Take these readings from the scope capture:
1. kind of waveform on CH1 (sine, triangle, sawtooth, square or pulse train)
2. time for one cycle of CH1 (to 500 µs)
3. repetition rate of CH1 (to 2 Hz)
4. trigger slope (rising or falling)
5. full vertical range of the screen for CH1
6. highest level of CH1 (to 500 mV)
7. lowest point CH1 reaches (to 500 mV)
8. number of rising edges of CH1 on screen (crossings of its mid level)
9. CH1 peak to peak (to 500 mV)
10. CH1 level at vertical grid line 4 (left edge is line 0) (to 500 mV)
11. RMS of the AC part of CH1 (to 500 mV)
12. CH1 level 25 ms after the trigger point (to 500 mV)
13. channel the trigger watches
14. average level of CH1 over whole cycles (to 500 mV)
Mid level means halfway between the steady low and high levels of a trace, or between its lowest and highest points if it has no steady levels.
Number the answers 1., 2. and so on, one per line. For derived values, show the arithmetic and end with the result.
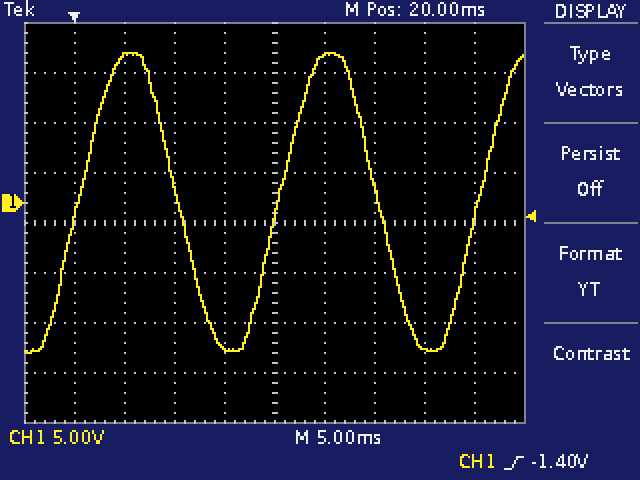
1. sine
2. 20.0 ms
3. 1 / 20.0 ms ≈ 50 Hz
4. rising
5. 40 V
6. 15.0 V
7. -15.0 V
8. 3
9. 15.0 V − (-15.0 V) = 30.0 V
10. -14.5 V
11. 30.0 V / (2√2) ≈ 10.6 V, so 10.5 V to the nearest 500 mV
12. 15.0 V
13. CH1
14. (15.0 V + (-15.0 V)) / 2 ≈ 0.0 V
